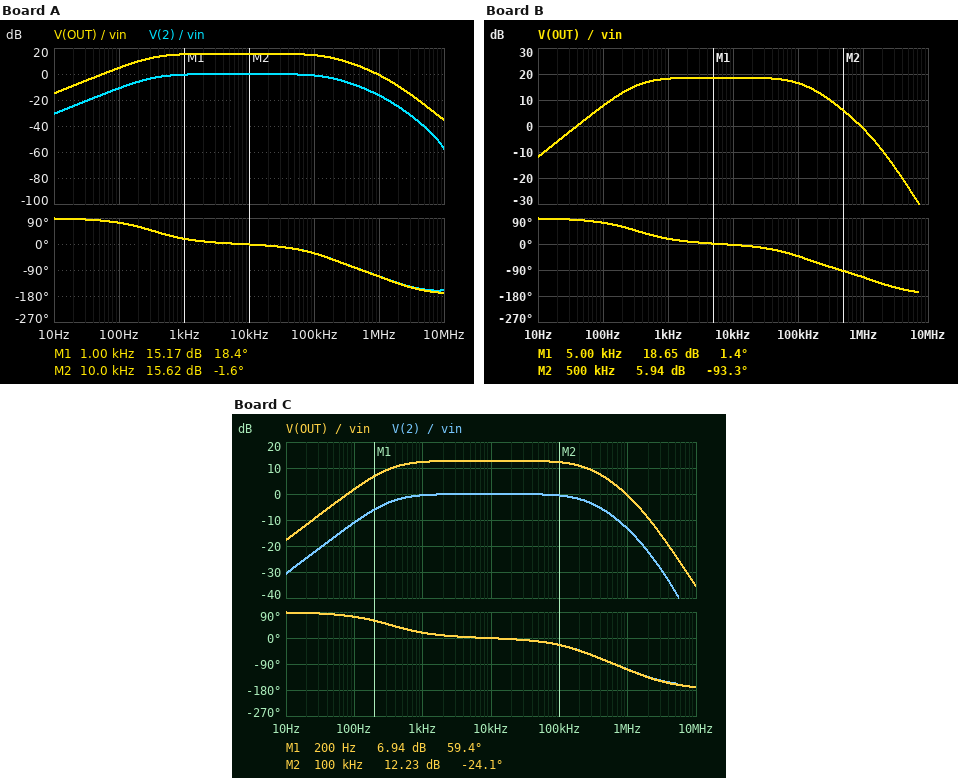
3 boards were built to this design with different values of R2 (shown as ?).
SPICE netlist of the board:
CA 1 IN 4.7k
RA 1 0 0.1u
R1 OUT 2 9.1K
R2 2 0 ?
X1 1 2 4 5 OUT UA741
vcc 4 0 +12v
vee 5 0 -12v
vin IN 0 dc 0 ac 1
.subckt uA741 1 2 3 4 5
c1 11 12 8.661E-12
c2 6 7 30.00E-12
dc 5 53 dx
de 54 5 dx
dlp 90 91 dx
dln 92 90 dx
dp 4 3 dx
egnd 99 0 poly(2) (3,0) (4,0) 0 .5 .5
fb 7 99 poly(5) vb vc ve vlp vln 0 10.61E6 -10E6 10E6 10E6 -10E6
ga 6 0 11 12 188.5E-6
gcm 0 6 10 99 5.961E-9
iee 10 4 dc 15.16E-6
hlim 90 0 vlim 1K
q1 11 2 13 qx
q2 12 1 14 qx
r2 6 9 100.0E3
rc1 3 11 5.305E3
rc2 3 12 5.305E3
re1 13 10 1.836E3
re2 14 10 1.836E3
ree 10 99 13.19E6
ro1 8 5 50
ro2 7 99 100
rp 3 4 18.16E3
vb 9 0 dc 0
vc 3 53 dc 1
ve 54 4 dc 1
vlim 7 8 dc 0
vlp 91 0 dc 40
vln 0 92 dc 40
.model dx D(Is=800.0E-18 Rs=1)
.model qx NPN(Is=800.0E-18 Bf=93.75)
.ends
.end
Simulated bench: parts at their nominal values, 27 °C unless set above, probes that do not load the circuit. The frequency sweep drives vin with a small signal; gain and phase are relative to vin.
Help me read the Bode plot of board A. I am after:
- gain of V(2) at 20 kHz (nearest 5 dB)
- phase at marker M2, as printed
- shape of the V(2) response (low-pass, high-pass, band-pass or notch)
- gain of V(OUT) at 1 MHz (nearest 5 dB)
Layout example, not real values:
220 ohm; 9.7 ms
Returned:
0 dB; -1.6 deg; band-pass; 0 dB
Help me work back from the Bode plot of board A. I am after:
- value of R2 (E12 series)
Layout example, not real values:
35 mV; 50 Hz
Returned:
1.8 kΩ
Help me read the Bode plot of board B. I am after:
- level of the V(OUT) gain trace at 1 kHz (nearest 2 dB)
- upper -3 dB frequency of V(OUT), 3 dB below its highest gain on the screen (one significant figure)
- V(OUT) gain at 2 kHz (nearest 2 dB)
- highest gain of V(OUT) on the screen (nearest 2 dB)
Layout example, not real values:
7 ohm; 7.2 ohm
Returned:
18 dB; 100 kHz; 18 dB; 18 dB
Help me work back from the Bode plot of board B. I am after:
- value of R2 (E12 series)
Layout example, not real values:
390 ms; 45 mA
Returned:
1.2 kΩ
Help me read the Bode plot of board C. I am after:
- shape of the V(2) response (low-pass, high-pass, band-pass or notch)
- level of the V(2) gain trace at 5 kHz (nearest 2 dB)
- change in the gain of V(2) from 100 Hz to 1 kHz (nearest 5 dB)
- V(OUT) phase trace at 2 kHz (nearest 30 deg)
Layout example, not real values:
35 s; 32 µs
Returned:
band-pass; 0 dB; 10 dB; 0 deg
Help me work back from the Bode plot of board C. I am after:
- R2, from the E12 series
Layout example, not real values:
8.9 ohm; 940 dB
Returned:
2.7 kΩ
